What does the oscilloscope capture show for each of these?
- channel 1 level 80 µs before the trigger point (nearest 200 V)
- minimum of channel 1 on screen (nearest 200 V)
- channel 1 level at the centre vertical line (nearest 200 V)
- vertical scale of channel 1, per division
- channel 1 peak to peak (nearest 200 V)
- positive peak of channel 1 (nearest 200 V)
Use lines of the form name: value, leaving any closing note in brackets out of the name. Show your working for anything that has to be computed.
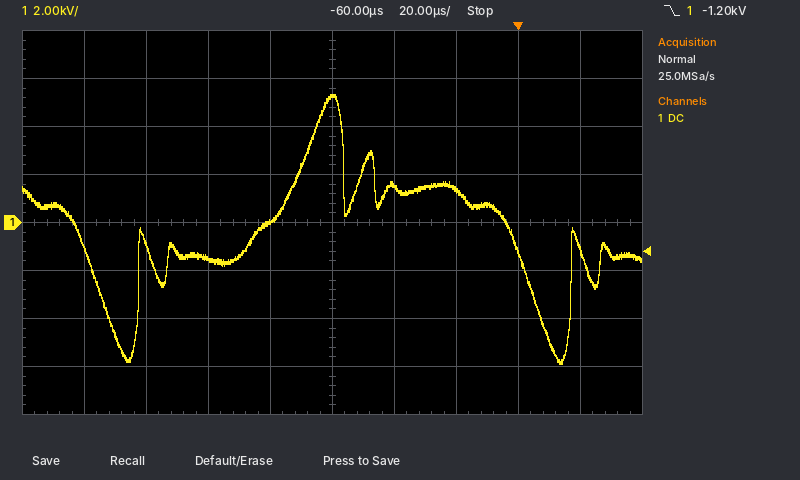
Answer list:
channel 1 level 80 µs before the trigger point: 0.0 kV
minimum of channel 1 on screen: -5.8 kV
channel 1 level at the centre vertical line: 5.2 kV
vertical scale of channel 1, per division: 2 kV
channel 1 peak to peak: 5.4 kV − (-5.8 kV) = 11.2 kV
positive peak of channel 1: 5.4 kV
